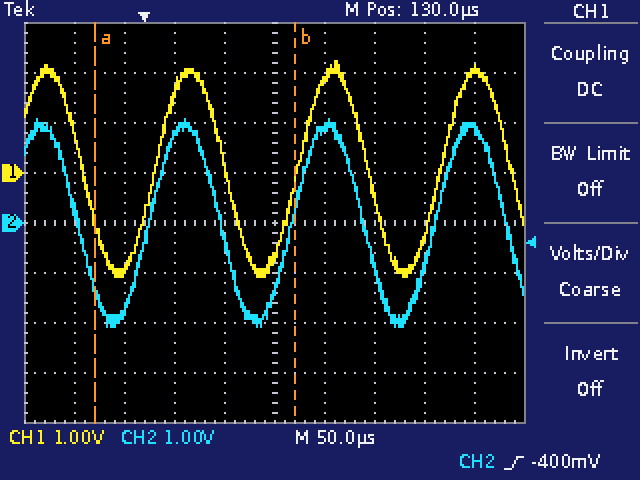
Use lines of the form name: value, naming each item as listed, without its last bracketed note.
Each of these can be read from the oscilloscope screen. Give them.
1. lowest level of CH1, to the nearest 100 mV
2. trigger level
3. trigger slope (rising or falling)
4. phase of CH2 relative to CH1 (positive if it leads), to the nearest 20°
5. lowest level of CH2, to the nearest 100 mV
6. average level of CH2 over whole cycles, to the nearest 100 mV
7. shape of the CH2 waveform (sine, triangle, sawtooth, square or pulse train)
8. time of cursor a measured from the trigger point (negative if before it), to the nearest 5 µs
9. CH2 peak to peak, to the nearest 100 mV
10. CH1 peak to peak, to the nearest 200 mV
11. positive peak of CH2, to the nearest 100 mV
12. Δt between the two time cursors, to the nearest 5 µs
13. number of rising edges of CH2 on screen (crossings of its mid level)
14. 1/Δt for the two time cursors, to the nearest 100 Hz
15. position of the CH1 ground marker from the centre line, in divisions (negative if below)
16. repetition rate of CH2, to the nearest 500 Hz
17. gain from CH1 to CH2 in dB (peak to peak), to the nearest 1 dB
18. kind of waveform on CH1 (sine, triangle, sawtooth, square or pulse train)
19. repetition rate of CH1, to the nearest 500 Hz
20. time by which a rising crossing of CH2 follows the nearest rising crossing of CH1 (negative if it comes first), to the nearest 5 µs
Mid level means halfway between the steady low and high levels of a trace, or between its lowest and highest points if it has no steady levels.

lowest level of CH1, to the nearest 100 mV: -2.1 V
trigger level: -400 mV
trigger slope: rising
phase of CH2 relative to CH1 (positive if it leads), to the nearest 20°: +20°
lowest level of CH2, to the nearest 100 mV: -2.1 V
average level of CH2 over whole cycles, to the nearest 100 mV: 0.0 V
shape of the CH2 waveform: sine
time of cursor a measured from the trigger point (negative if before it), to the nearest 5 µs: -50 µs
CH2 peak to peak, to the nearest 100 mV: 4.2 V
CH1 peak to peak, to the nearest 200 mV: 4.4 V
positive peak of CH2, to the nearest 100 mV: 2.1 V
Δt between the two time cursors, to the nearest 5 µs: 200 µs
number of rising edges of CH2 on screen: 3
1/Δt for the two time cursors, to the nearest 100 Hz: 5.0 kHz
position of the CH1 ground marker from the centre line, in divisions: +1.0 div
repetition rate of CH2, to the nearest 500 Hz: 7.0 kHz
gain from CH1 to CH2 in dB (peak to peak), to the nearest 1 dB: 0 dB
kind of waveform on CH1: sine
repetition rate of CH1, to the nearest 500 Hz: 7.0 kHz
time by which a rising crossing of CH2 follows the nearest rising crossing of CH1 (negative if it comes first), to the nearest 5 µs: -5 µs
